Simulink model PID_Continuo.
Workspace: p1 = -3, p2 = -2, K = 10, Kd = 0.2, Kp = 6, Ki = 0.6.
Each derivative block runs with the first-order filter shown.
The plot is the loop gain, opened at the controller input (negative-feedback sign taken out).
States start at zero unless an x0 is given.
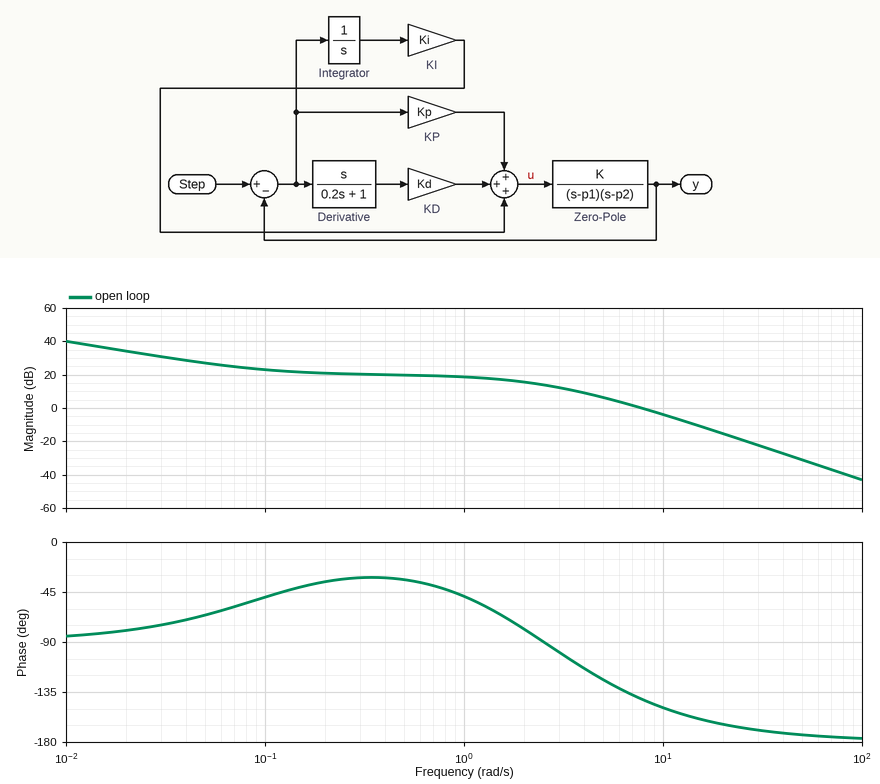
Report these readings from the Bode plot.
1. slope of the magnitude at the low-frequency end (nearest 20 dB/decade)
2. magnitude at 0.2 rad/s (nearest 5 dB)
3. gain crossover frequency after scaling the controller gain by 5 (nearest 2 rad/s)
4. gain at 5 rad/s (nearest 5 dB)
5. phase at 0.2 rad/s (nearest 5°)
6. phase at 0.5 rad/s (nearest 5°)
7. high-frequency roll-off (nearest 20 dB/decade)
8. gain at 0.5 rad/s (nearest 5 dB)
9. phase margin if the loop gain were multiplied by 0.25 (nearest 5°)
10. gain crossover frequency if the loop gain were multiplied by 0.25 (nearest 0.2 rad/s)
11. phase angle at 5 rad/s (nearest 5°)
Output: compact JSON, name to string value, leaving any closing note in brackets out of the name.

{"slope of the magnitude at the low-frequency end": "-20 dB/decade", "magnitude at 0.2 rad/s": "20 dB", "gain crossover frequency after scaling the controller gain by 5": "18 rad/s", "gain at 5 rad/s": "5 dB", "phase at 0.2 rad/s": "-35°", "phase at 0.5 rad/s": "-35°", "high-frequency roll-off": "-40 dB/decade", "gain at 0.5 rad/s": "20 dB", "phase margin if the loop gain were multiplied by 0.25": "80°", "gain crossover frequency if the loop gain were multiplied by 0.25": "3.0 rad/s", "phase angle at 5 rad/s": "-125°"}
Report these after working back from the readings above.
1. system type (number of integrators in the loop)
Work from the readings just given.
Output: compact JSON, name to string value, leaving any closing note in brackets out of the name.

{"system type": "1"}
